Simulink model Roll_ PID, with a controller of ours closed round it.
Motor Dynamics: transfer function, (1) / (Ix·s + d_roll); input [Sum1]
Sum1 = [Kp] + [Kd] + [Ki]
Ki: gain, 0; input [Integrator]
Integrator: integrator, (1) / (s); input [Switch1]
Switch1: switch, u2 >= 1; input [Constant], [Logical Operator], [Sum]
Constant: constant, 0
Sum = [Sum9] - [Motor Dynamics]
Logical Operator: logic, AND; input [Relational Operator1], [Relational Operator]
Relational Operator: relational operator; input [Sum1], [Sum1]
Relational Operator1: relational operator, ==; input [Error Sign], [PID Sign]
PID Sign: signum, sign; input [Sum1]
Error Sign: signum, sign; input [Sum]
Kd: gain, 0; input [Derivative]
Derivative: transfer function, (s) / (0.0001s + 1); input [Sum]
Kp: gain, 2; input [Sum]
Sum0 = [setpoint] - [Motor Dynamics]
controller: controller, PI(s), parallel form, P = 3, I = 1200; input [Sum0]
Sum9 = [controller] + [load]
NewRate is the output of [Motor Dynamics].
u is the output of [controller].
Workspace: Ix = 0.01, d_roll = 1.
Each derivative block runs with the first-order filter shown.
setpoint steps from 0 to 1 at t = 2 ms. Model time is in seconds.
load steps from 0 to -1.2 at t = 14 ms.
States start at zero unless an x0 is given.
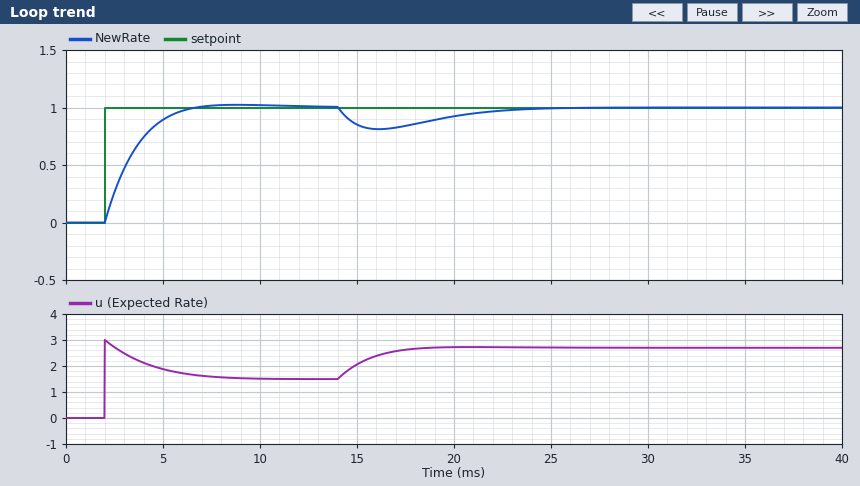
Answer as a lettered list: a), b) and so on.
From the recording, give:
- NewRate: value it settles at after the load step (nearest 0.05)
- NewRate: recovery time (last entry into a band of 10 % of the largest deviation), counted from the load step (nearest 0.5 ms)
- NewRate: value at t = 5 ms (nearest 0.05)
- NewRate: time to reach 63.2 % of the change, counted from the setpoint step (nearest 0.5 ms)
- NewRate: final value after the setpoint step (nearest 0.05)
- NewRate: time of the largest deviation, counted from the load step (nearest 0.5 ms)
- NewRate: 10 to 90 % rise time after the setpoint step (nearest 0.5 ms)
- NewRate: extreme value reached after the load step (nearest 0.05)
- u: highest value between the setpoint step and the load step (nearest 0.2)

a) 1.00
b) 9.0 ms
c) 0.90
d) 1.5 ms
e) 1.00
f) 2.0 ms
g) 3.0 ms
h) 0.80
i) 3.0
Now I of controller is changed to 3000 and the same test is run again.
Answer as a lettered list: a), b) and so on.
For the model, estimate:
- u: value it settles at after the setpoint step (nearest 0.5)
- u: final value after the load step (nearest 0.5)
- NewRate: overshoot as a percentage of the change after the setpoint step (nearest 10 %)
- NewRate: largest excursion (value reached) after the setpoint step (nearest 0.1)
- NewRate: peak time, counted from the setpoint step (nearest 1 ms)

a) 1.5
b) 2.5
c) 20 %
d) 1.2
e) 4 ms
